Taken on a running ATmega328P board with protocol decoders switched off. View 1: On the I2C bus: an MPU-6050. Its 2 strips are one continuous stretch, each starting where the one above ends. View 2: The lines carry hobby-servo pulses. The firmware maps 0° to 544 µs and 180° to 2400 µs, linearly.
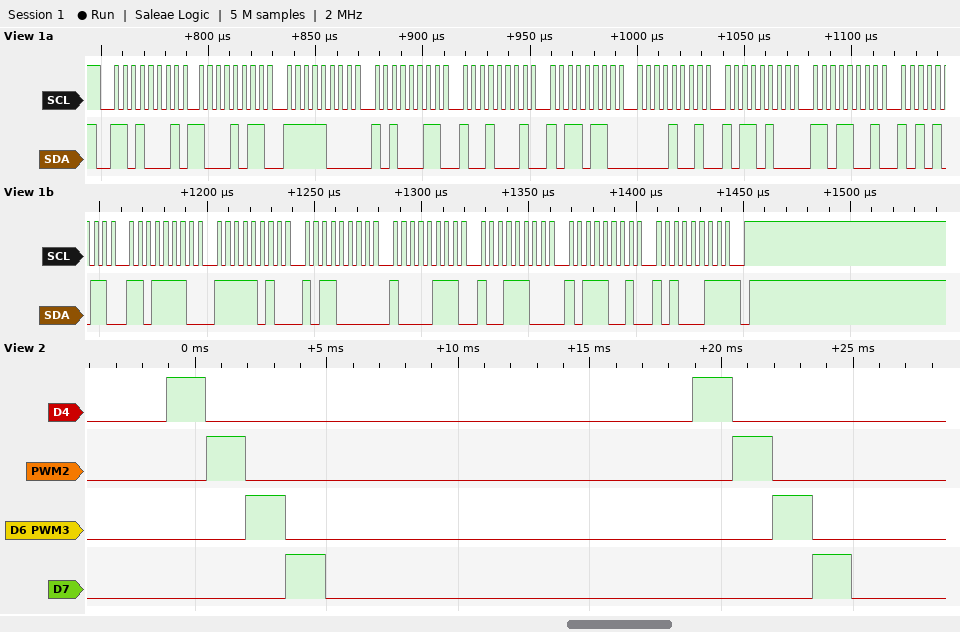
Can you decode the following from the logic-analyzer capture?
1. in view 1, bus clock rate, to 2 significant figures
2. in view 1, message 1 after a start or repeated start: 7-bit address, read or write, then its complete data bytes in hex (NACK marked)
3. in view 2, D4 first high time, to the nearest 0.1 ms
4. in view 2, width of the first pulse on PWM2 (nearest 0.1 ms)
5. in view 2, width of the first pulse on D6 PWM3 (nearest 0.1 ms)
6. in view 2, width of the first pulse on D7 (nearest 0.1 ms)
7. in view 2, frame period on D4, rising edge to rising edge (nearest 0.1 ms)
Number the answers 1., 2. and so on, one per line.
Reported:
1. 250 kHz
2. 0x68 read: 8B F8 A3 91 B6 09 B4 D9 AB DE FA B0 87 9C B9 A3 NACK
3. 1.5 ms
4. 1.5 ms
5. 1.5 ms
6. 1.5 ms
7. 20.0 ms
